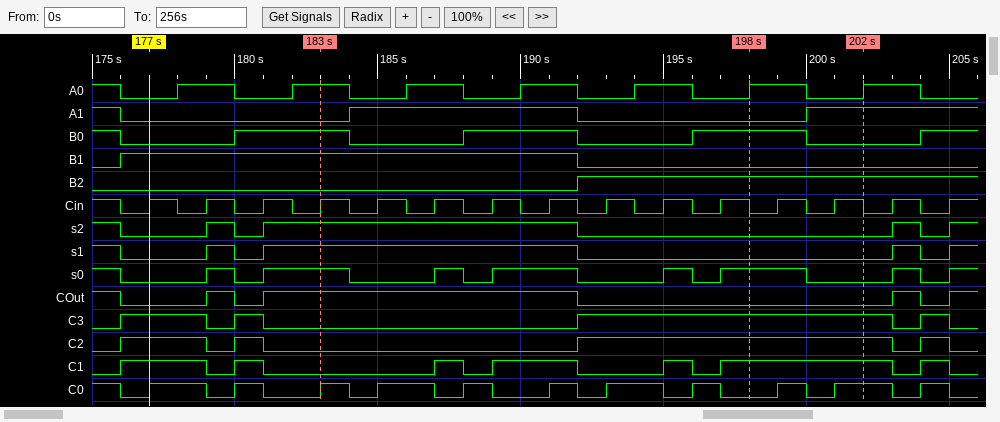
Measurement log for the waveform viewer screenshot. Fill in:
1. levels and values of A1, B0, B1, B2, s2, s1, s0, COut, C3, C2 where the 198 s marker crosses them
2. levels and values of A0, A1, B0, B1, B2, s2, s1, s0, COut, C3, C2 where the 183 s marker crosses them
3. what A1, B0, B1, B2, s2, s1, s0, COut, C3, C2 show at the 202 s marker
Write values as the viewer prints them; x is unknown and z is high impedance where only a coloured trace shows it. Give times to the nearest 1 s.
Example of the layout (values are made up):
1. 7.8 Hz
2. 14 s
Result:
1. A1=0, B0=1, B1=0, B2=1, s2=0, s1=0, s0=1, COut=0, C3=1, C2=1
2. A0=1, A1=0, B0=1, B1=1, B2=0, s2=1, s1=1, s0=1, COut=1, C3=0, C2=0
3. A1=1, B0=0, B1=0, B2=1, s2=0, s1=0, s0=0, COut=0, C3=1, C2=1
